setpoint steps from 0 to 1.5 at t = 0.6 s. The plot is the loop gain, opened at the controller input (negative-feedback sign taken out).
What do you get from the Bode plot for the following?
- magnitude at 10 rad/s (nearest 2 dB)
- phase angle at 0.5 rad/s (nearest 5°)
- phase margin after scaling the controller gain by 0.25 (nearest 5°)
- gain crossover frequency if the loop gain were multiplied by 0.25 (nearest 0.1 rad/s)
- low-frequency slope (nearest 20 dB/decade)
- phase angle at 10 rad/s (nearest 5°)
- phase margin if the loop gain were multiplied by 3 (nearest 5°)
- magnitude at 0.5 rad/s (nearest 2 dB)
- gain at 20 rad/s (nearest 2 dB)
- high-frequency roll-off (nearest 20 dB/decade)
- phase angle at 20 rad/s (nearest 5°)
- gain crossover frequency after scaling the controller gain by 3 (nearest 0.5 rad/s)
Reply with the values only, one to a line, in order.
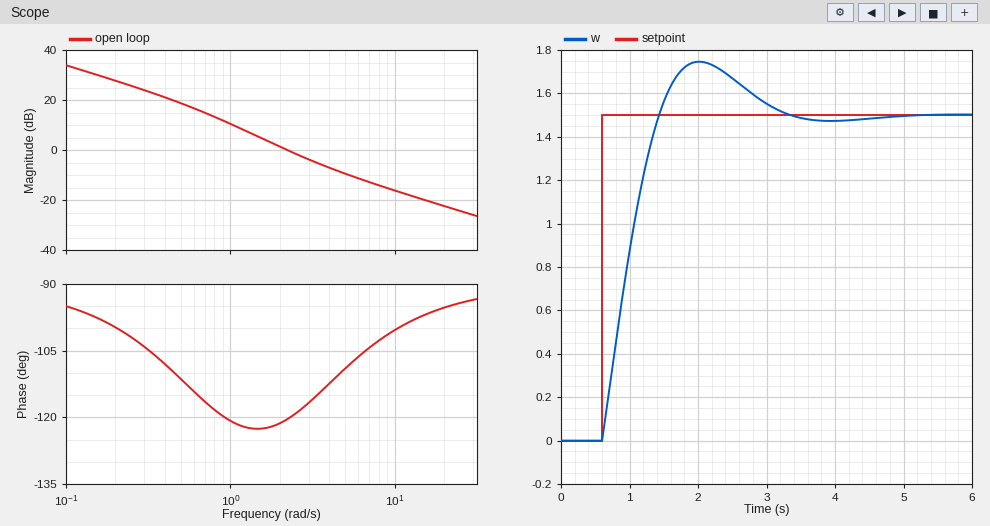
-16 dB
-110°
60°
0.9 rad/s
-20 dB/decade
-100°
70°
18 dB
-22 dB
-20 dB/decade
-95°
5.0 rad/s
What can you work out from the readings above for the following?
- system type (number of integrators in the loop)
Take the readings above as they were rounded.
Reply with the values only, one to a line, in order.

1
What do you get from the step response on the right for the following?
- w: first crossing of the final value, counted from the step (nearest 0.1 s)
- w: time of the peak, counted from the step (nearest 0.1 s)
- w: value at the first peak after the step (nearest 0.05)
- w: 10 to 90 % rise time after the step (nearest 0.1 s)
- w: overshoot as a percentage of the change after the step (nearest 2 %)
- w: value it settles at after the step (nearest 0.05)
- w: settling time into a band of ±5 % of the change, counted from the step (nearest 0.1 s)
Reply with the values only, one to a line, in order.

0.8 s
1.4 s
1.75
0.6 s
16 %
1.50
2.3 s
